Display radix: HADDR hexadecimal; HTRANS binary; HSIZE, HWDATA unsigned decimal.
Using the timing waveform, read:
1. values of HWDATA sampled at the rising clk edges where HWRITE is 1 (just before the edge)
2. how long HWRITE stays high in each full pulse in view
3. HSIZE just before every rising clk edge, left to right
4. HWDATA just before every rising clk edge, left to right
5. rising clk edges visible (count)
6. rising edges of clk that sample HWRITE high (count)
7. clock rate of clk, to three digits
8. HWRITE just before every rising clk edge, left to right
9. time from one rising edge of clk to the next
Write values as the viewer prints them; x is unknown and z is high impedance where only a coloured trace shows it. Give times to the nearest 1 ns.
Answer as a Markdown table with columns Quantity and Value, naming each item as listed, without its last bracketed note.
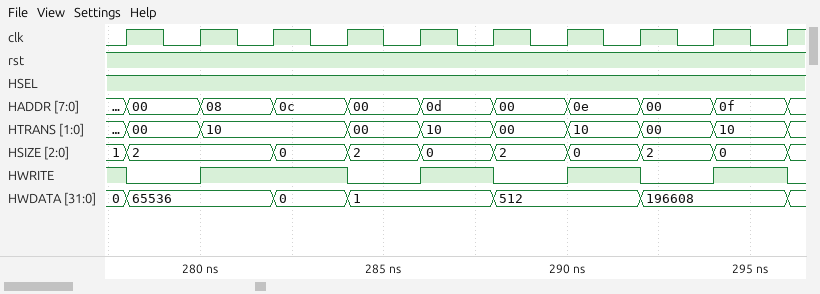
| Quantity | Value |
|---|---|
| values of HWDATA sampled at the rising clk edges where HWRITE is 1 | 0, 65536, 0, 1, 512, 196608 |
| how long HWRITE stays high in each full pulse in view | 4 ns, 2 ns, 2 ns, 2 ns |
| HSIZE just before every rising clk edge, left to right | 1, 2, 2, 0, 2, 0, 2, 0, 2, 0 |
| HWDATA just before every rising clk edge, left to right | 0, 65536, 65536, 0, 1, 1, 512, 512, 196608, 196608 |
| rising clk edges visible | 10 |
| rising edges of clk that sample HWRITE high | 6 |
| clock rate of clk, to three digits | 500 MHz |
| HWRITE just before every rising clk edge, left to right | 1 0 1 1 0 1 0 1 0 1 |
| time from one rising edge of clk to the next | 2 ns |
